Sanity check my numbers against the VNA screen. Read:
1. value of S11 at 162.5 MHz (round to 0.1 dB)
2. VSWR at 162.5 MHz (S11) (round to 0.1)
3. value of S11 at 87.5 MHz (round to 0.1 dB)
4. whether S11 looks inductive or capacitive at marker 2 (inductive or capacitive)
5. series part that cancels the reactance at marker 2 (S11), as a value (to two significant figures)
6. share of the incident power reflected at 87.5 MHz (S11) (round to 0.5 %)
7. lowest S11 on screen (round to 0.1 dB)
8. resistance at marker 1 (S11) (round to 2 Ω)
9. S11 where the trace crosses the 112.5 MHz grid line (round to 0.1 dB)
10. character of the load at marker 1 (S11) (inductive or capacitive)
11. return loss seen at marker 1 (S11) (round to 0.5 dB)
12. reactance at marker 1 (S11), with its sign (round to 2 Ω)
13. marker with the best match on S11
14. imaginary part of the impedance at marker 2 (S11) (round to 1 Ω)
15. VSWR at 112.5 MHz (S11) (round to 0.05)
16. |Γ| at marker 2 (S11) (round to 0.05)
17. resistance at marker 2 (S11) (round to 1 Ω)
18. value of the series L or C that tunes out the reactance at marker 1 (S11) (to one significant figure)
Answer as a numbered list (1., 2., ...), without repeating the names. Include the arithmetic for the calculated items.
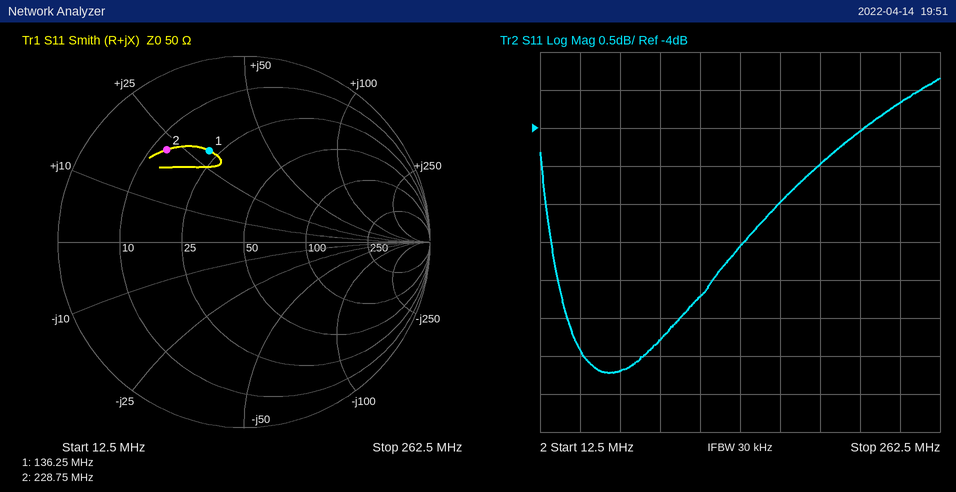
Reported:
1. -5.0 dB
2. |Γ| = 10^(-5/20) = 0.5623; VSWR = (1 + 0.5623)/(1 − 0.5623) ≈ 3.6
3. -6.8 dB
4. inductive
5. C = 1/(2π × 228.75 MHz × 22 Ω) ≈ 32 pF
6. 10^(-6.8/10) ≈ 20.9 %, so 21.0 % to the nearest 0.5 %
7. -7.2 dB
8. 22 Ω
9. -6.2 dB
10. inductive
11. 5.5 dB
12. +30 Ω
13. marker 1
14. +22 Ω
15. |Γ| = 10^(-6.2/20) = 0.4898; VSWR = (1 + 0.4898)/(1 − 0.4898) ≈ 2.92, so 2.90 to the nearest 0.05
16. 0.65
17. 13 Ω
18. C = 1/(2π × 136.25 MHz × 30 Ω) ≈ 38.9 pF, so 40 pF to one significant figure
